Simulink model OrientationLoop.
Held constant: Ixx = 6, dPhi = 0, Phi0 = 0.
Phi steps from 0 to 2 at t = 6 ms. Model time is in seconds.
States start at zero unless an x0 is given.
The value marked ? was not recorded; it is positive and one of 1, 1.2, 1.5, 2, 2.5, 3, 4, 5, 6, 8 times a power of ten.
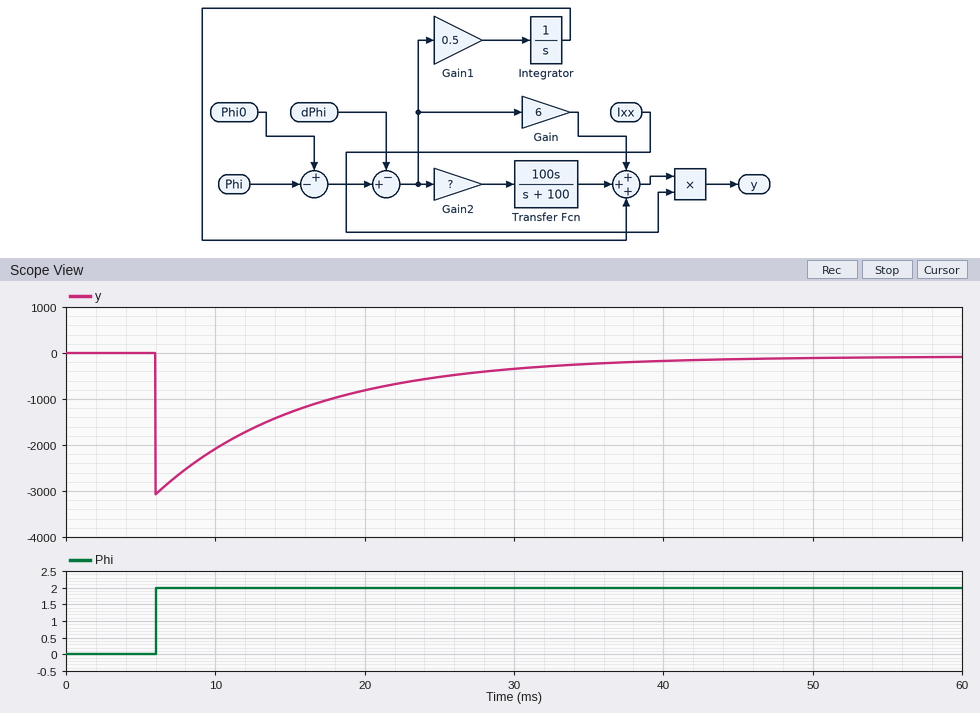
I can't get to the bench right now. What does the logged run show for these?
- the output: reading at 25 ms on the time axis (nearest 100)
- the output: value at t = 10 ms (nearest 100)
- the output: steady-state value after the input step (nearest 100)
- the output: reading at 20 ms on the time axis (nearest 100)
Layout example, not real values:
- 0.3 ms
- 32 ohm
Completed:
- -500
- -2100
- -100
- -800
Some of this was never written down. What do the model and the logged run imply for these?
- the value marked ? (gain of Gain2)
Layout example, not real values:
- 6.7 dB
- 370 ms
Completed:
- 2.5
